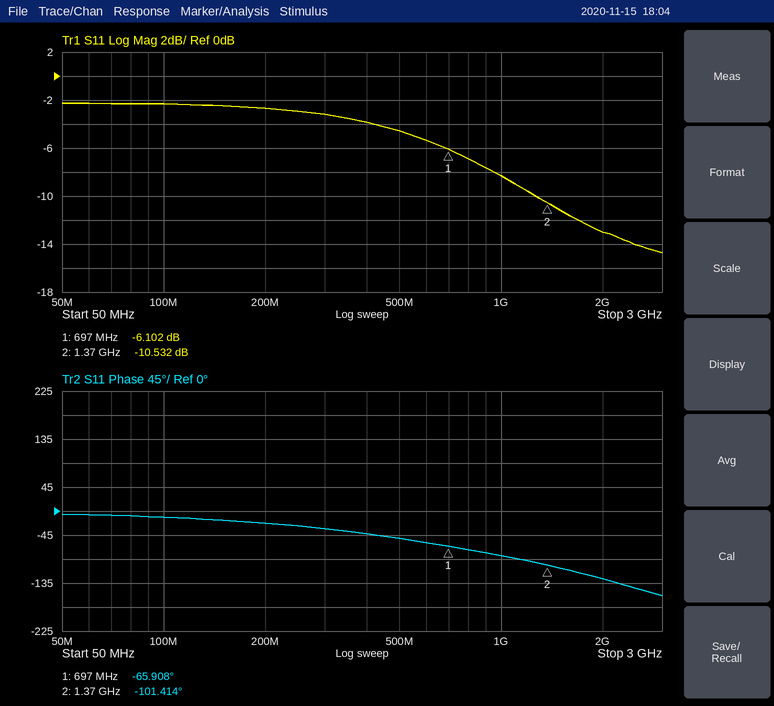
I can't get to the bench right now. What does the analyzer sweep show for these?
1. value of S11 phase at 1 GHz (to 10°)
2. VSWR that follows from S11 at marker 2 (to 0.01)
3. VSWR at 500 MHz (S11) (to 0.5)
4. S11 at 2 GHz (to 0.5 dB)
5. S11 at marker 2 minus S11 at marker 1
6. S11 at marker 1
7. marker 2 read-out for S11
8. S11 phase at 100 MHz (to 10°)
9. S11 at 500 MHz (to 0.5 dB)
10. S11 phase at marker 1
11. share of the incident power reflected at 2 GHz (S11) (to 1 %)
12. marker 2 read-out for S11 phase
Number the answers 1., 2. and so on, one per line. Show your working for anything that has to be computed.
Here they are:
1. -80°
2. (1 + 0.2974)/(1 − 0.2974) ≈ 1.85
3. |Γ| = 10^(-4.5/20) = 0.5957; VSWR = (1 + 0.5957)/(1 − 0.5957) ≈ 4.0
4. -13.0 dB
5. -10.532 − (-6.102) = -4.430 dB
6. -6.102 dB
7. -10.532 dB
8. -10°
9. -4.5 dB
10. -65.908°
11. 10^(-13/10) ≈ 5 %
12. -101.414°
